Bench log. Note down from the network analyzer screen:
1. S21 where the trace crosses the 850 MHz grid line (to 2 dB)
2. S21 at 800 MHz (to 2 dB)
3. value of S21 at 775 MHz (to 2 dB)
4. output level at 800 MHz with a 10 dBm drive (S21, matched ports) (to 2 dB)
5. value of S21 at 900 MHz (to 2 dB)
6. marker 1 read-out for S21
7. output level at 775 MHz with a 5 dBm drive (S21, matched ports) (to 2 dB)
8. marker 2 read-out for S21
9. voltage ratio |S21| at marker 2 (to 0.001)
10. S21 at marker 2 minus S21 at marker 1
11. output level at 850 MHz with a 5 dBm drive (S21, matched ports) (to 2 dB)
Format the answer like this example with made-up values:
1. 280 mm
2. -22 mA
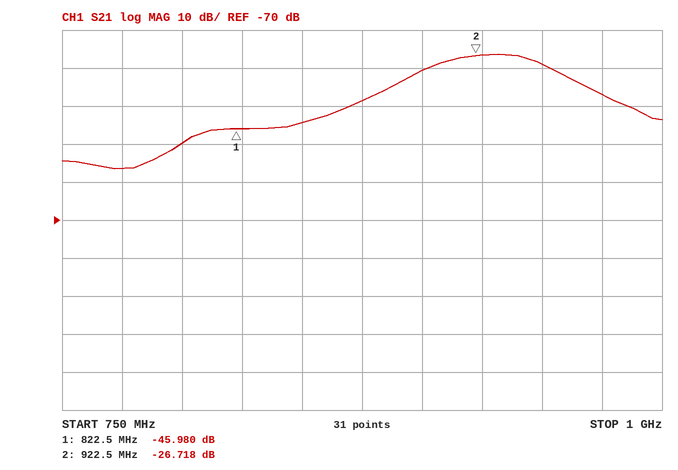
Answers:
1. -44 dB
2. -50 dB
3. -56 dB
4. -40 dBm
5. -30 dB
6. -45.980 dB
7. -52 dBm
8. -26.718 dB
9. 0.046
10. 19.262 dB
11. -40 dBm
